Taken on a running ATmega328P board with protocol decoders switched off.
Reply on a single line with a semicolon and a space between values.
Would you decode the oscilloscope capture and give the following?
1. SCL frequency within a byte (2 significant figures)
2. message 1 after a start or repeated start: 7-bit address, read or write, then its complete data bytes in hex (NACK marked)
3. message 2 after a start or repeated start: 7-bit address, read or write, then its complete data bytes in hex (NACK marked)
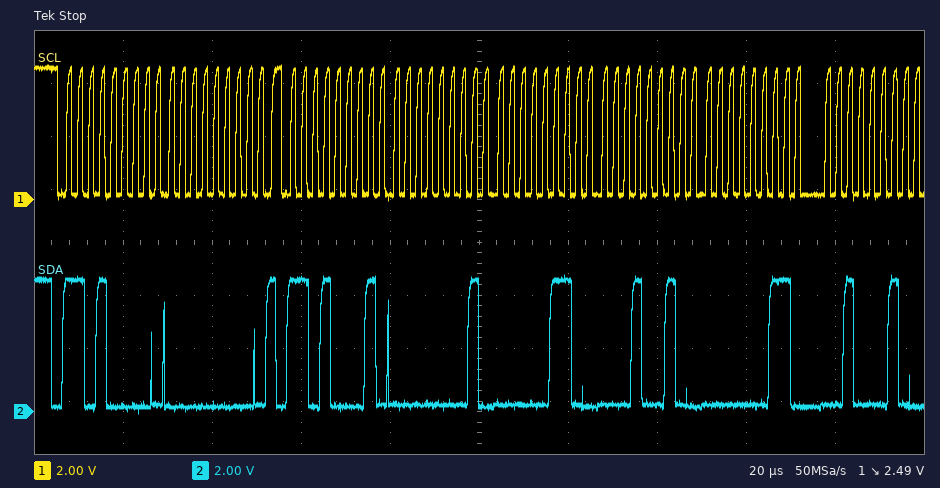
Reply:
400 kHz; 0x68 write: 00; 0x68 read: 01 06 12 03 22
